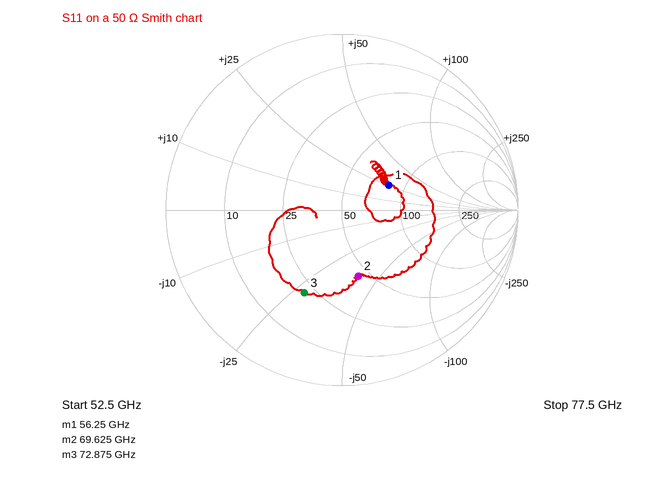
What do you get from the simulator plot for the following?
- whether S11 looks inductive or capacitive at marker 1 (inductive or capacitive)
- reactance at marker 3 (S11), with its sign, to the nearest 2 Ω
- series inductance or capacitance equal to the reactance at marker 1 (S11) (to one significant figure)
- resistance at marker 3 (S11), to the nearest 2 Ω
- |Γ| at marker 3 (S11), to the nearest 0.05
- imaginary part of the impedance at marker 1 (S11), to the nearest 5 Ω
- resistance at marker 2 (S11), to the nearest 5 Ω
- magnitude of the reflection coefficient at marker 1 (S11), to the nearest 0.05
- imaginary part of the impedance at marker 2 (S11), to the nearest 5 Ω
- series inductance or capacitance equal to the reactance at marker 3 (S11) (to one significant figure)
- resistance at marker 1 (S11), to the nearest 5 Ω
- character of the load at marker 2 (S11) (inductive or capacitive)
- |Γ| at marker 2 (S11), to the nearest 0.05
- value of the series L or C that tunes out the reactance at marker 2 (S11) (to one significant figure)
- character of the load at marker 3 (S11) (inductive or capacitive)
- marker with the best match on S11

inductive
-28 Ω
70 pH
22 Ω
0.50
+25 Ω
45 Ω
0.30
-40 Ω
80 fF
80 Ω
capacitive
0.40
90 pH
capacitive
marker 1
